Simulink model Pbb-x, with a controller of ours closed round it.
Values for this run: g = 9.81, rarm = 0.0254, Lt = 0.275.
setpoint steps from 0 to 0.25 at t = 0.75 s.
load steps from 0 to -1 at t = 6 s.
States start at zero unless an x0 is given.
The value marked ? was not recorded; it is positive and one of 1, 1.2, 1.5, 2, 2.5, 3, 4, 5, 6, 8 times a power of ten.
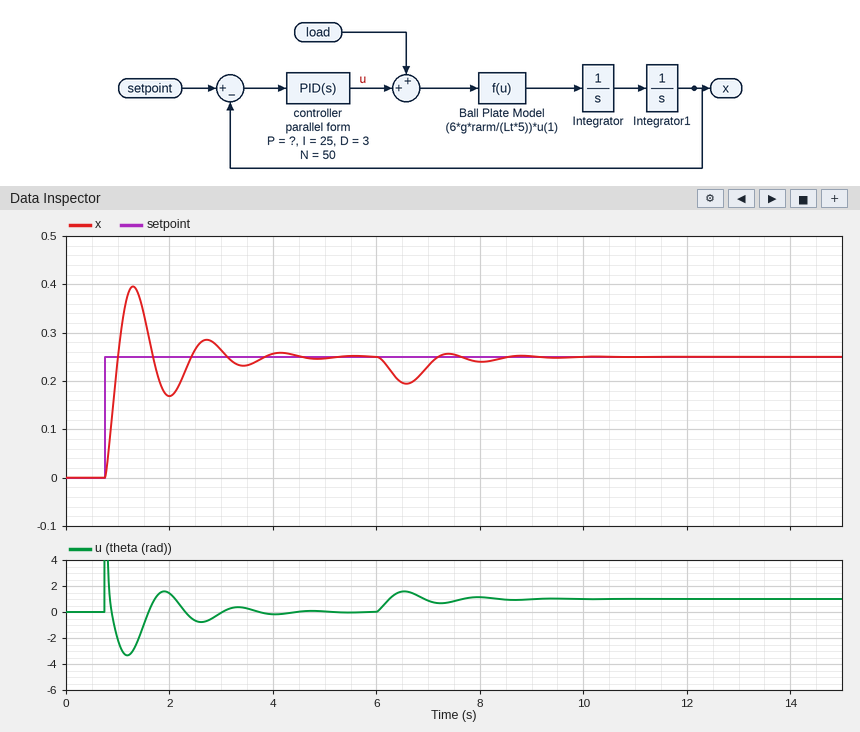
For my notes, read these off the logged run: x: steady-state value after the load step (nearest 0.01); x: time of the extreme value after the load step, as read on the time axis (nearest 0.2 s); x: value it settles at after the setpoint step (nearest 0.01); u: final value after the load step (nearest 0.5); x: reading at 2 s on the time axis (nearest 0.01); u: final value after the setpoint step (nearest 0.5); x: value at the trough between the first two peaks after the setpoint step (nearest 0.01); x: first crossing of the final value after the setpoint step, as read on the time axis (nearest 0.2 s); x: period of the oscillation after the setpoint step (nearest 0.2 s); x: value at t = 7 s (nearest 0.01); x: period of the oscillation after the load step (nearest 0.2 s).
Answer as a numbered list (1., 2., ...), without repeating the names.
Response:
1. 0.25
2. 6.6 s
3. 0.25
4. 1.0
5. 0.17
6. 0.0
7. 0.17
8. 1.0 s
9. 1.4 s
10. 0.23
11. 1.4 s
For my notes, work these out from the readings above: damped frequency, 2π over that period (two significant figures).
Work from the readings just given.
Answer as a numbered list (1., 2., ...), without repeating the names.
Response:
1. 4.5 rad/s
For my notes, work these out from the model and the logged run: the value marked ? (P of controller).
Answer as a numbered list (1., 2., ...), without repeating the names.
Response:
1. 20
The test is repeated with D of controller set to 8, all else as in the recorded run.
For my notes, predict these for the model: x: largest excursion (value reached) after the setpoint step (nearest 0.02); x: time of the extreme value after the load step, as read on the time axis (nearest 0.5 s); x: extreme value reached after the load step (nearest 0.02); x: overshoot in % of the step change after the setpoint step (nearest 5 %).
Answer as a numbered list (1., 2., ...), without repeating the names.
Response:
1. 0.30
2. 6.5 s
3. 0.22
4. 20 %
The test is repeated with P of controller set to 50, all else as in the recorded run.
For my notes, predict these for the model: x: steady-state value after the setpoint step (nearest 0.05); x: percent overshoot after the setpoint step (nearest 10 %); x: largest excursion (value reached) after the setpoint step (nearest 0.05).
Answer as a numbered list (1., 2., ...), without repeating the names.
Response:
1. 0.25
2. 60 %
3. 0.40
